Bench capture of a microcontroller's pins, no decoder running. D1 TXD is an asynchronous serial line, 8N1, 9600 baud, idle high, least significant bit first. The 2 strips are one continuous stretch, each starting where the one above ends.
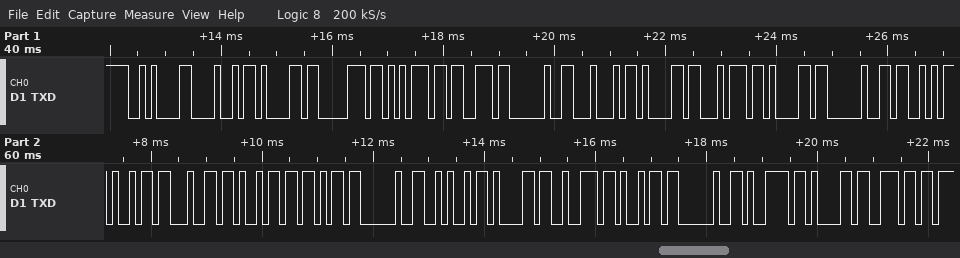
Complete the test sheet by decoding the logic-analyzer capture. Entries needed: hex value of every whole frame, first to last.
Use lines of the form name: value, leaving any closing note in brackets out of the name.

hex value of every whole frame, first to last: 0A 48 61 70 75 73 20 44 61 74 61 20 53 69 64 69 6B 20 4A 61 72 69 20 79 61 6E
